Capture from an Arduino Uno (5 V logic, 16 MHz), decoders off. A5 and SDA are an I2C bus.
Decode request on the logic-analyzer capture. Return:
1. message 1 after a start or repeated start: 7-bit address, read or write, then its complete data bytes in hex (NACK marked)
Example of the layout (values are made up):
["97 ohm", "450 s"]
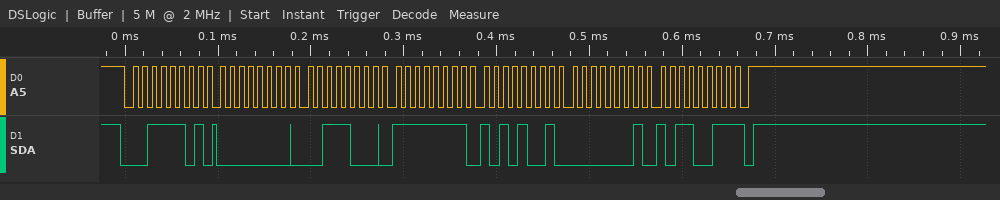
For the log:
["0x1E read: 00 38 FF A9 01 B3 NACK"]
